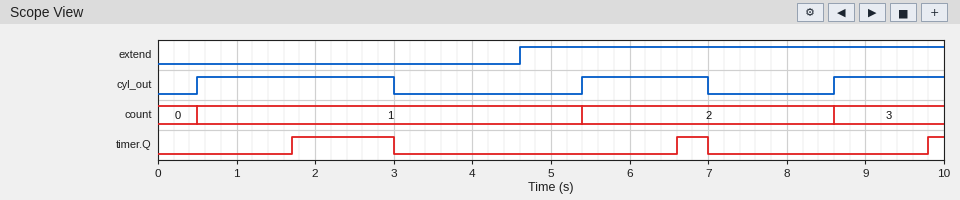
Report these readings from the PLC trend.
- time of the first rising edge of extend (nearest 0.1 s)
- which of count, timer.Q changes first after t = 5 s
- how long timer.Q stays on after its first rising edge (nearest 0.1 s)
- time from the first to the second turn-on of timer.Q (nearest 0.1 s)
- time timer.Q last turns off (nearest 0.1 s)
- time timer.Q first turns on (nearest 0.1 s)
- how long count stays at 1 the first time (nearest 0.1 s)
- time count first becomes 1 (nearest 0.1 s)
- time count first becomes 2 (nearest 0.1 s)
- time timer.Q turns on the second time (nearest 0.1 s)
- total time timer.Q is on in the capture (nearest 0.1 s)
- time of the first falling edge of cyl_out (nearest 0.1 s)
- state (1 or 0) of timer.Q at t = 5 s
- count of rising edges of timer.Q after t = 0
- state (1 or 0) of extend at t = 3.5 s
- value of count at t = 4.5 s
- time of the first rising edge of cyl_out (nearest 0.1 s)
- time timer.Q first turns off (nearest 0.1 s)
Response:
4.6 s
count
1.3 s
4.9 s
7.0 s
1.7 s
4.9 s
0.5 s
5.4 s
6.6 s
1.9 s
3.0 s
0
3
0
1
0.5 s
3.0 s
